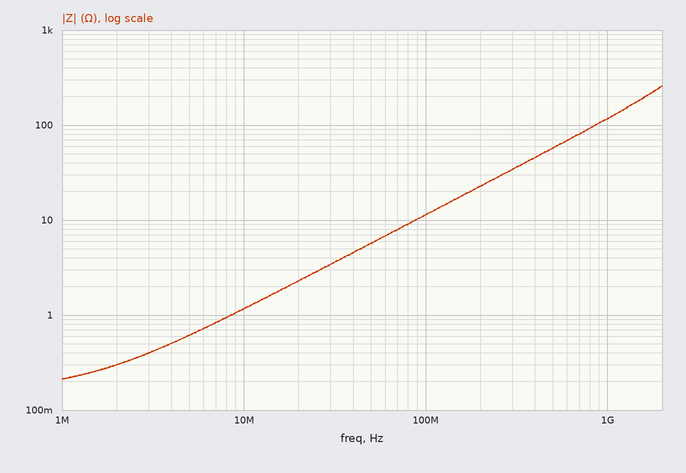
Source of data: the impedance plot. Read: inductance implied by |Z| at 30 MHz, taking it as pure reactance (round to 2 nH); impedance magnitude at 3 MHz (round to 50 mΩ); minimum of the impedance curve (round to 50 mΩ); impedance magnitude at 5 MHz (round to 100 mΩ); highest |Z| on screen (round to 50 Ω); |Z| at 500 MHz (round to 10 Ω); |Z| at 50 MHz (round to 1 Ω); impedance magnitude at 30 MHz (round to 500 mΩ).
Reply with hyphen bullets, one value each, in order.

- 18 nH
- 400 mΩ
- 200 mΩ
- 600 mΩ
- 250 Ω
- 60 Ω
- 6 Ω
- 3.5 Ω
